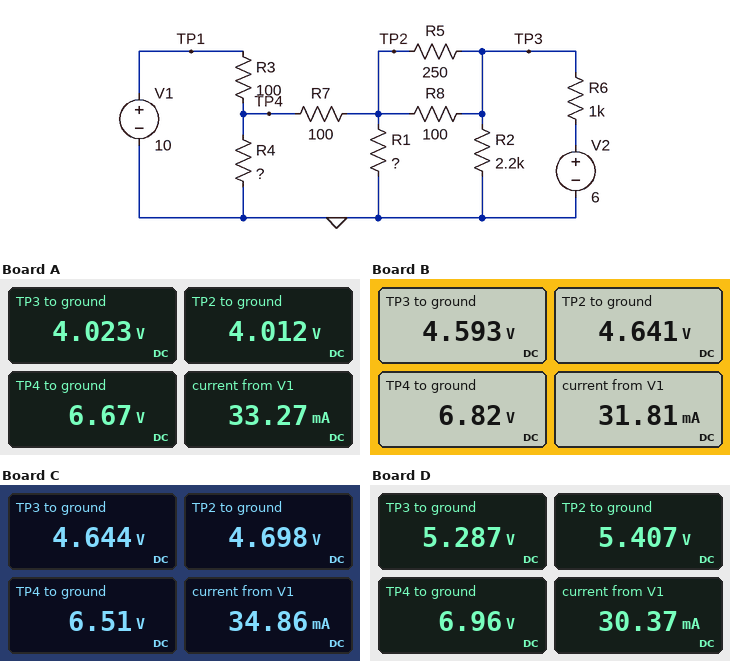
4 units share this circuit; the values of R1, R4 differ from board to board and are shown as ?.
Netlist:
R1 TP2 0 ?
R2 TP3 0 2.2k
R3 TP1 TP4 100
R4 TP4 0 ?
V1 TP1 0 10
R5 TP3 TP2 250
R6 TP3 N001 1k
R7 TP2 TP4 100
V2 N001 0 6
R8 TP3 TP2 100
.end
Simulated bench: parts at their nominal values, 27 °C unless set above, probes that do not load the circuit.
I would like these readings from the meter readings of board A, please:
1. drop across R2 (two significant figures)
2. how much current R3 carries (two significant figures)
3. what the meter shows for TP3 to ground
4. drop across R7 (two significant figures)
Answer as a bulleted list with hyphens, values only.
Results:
- 4.0 V
- 33 mA
- 4.023 V
- 2.7 V
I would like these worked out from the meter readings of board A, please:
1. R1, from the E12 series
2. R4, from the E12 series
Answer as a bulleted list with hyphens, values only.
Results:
- 150 Ω
- 1 kΩ
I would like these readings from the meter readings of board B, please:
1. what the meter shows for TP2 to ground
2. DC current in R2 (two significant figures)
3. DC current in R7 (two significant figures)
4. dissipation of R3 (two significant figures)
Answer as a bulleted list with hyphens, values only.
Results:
- 4.641 V
- 2.1 mA
- 22 mA
- 100 mW
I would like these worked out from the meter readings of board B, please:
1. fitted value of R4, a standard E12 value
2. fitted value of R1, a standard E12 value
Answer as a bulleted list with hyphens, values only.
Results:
- 680 Ω
- 220 Ω
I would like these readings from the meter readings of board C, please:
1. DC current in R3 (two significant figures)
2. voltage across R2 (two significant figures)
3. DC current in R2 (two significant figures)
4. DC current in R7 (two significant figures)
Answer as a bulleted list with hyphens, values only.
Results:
- 35 mA
- 4.6 V
- 2.1 mA
- 18 mA
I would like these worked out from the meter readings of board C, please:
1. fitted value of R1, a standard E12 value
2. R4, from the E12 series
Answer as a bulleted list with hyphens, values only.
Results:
- 270 Ω
- 390 Ω
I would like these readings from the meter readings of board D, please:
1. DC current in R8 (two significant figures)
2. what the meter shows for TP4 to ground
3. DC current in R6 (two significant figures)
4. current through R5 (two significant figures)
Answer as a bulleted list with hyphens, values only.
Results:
- 1.2 mA
- 6.96 V
- 710 µA
- 480 µA
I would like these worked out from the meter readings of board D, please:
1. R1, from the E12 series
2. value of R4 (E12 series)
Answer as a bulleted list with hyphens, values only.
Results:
- 390 Ω
- 470 Ω
